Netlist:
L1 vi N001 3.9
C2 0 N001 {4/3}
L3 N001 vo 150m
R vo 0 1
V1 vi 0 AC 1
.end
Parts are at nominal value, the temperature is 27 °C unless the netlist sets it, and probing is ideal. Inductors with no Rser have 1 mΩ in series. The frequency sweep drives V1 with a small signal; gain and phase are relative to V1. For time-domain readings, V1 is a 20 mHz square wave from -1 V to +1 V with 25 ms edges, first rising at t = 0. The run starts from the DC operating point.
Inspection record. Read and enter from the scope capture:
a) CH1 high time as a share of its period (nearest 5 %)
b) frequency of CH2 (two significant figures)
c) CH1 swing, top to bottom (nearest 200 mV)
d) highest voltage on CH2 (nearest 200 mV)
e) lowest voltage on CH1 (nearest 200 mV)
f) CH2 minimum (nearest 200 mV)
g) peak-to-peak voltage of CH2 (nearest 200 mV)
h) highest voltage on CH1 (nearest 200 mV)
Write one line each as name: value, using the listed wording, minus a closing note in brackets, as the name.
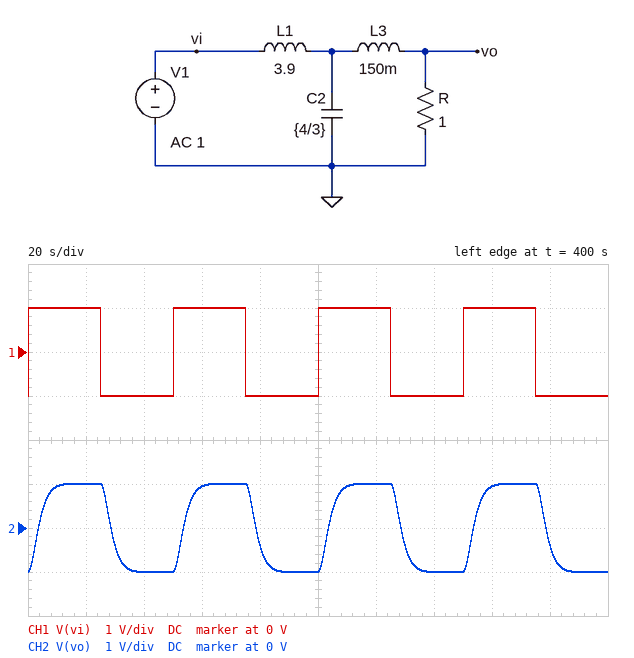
CH1 high time as a share of its period: 50 %
frequency of CH2: 20 mHz
CH1 swing, top to bottom: 2.0 V
highest voltage on CH2: 1.0 V
lowest voltage on CH1: -1.0 V
CH2 minimum: -1.0 V
peak-to-peak voltage of CH2: 2.0 V
highest voltage on CH1: 1.0 V
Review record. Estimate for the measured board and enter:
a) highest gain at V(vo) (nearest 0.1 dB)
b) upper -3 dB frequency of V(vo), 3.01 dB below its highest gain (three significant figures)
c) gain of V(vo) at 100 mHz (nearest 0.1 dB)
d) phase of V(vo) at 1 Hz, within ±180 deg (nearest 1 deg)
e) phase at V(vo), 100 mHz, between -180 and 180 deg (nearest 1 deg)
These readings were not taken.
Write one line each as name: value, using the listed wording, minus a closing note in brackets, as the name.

highest gain at V(vo): 0 dB
upper -3 dB frequency of V(vo), 3.01 dB below its highest gain: 54.8 mHz
gain of V(vo) at 100 mHz: -8.2 dB
phase of V(vo) at 1 Hz, within ±180 deg: 141 deg
phase at V(vo), 100 mHz, between -180 and 180 deg: -114 deg
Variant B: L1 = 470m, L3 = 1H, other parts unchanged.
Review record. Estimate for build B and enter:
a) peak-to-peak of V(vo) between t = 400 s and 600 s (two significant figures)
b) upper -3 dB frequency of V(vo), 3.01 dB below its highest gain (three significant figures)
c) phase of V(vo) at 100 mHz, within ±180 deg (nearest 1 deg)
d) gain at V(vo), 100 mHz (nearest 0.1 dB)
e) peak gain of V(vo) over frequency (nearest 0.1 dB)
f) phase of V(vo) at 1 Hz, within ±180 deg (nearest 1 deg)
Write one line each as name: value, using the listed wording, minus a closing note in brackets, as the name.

peak-to-peak of V(vo) between t = 400 s and 600 s: 2.9 V
upper -3 dB frequency of V(vo), 3.01 dB below its highest gain: 249 mHz
phase of V(vo) at 100 mHz, within ±180 deg: -46 deg
gain at V(vo), 100 mHz: -0.6 dB
peak gain of V(vo) over frequency: 8.2 dB
phase of V(vo) at 1 Hz, within ±180 deg: 99 deg
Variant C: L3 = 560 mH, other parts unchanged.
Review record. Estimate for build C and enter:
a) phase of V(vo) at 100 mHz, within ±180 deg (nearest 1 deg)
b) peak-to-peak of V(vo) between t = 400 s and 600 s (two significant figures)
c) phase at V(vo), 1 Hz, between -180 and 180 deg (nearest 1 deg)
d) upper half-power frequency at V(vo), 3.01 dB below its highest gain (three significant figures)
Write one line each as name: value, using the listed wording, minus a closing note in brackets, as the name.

phase of V(vo) at 100 mHz, within ±180 deg: -117 deg
peak-to-peak of V(vo) between t = 400 s and 600 s: 2.0 V
phase at V(vo), 1 Hz, between -180 and 180 deg: 106 deg
upper half-power frequency at V(vo), 3.01 dB below its highest gain: 51.3 mHz
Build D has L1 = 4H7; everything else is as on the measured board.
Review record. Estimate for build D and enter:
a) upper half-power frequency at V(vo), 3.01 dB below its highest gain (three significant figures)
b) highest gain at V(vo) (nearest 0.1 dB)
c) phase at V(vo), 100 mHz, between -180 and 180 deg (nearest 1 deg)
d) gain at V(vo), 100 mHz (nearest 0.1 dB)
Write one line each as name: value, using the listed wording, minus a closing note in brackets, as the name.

upper half-power frequency at V(vo), 3.01 dB below its highest gain: 43.8 mHz
highest gain at V(vo): 0 dB
phase at V(vo), 100 mHz, between -180 and 180 deg: -118 deg
gain at V(vo), 100 mHz: -10.0 dB
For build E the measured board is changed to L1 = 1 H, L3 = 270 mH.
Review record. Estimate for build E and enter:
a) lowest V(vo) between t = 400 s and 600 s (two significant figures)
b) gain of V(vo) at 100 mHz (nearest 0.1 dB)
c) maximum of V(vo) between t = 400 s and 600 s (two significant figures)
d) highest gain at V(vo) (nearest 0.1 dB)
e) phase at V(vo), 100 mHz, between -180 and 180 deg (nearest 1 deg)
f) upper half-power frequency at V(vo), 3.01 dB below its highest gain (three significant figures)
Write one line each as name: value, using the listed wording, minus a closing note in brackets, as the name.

lowest V(vo) between t = 400 s and 600 s: -1.4 V
gain of V(vo) at 100 mHz: 1.4 dB
maximum of V(vo) between t = 400 s and 600 s: 1.4 V
highest gain at V(vo): 1.5 dB
phase at V(vo), 100 mHz, between -180 and 180 deg: -56 deg
upper half-power frequency at V(vo), 3.01 dB below its highest gain: 183 mHz
